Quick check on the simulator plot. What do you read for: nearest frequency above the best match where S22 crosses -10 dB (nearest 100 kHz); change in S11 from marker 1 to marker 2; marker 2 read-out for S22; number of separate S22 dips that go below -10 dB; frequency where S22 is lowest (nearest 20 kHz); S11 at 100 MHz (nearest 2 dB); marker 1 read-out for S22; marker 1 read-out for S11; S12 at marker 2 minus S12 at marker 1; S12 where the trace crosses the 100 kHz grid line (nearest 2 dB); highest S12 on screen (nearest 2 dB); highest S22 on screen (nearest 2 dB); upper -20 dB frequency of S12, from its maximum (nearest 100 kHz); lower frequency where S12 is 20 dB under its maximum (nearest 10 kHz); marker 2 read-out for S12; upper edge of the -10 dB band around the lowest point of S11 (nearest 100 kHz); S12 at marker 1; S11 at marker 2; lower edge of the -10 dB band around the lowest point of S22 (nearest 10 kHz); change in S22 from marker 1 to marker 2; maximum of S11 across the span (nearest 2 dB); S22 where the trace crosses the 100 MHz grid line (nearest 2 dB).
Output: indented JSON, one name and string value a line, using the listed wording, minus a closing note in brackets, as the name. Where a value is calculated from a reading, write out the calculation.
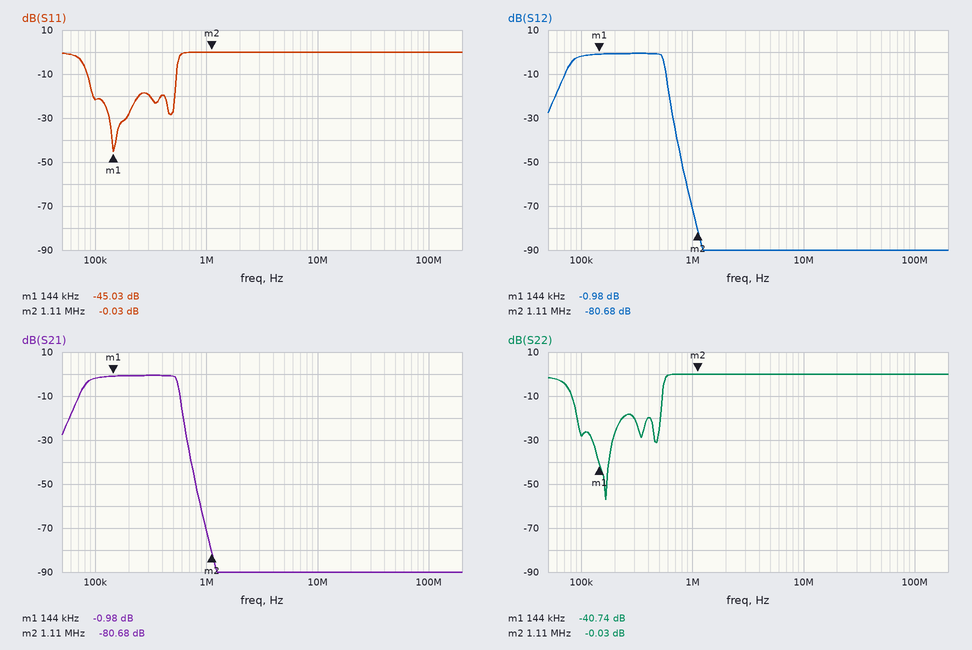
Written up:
{
  "nearest frequency above the best match where S22 crosses -10 dB": "500 kHz",
  "change in S11 from marker 1 to marker 2": "-0.03 − (-45.03) = 45.00 dB",
  "marker 2 read-out for S22": "-0.03 dB",
  "number of separate S22 dips that go below -10 dB": "3",
  "frequency where S22 is lowest": "160 kHz",
  "S11 at 100 MHz": "0 dB",
  "marker 1 read-out for S22": "-40.74 dB",
  "marker 1 read-out for S11": "-45.03 dB",
  "S12 at marker 2 minus S12 at marker 1": "-80.68 − (-0.98) = -79.70 dB",
  "S12 where the trace crosses the 100 kHz grid line": "-2 dB",
  "highest S12 on screen": "0 dB",
  "highest S22 on screen": "0 dB",
  "upper -20 dB frequency of S12, from its maximum": "600 kHz",
  "lower frequency where S12 is 20 dB under its maximum": "60 kHz",
  "marker 2 read-out for S12": "-80.68 dB",
  "upper edge of the -10 dB band around the lowest point of S11": "500 kHz",
  "S12 at marker 1": "-0.98 dB",
  "S11 at marker 2": "-0.03 dB",
  "lower edge of the -10 dB band around the lowest point of S22": "80 kHz",
  "change in S22 from marker 1 to marker 2": "-0.03 − (-40.74) = 40.71 dB",
  "maximum of S11 across the span": "0 dB",
  "S22 where the trace crosses the 100 MHz grid line": "0 dB"
}
